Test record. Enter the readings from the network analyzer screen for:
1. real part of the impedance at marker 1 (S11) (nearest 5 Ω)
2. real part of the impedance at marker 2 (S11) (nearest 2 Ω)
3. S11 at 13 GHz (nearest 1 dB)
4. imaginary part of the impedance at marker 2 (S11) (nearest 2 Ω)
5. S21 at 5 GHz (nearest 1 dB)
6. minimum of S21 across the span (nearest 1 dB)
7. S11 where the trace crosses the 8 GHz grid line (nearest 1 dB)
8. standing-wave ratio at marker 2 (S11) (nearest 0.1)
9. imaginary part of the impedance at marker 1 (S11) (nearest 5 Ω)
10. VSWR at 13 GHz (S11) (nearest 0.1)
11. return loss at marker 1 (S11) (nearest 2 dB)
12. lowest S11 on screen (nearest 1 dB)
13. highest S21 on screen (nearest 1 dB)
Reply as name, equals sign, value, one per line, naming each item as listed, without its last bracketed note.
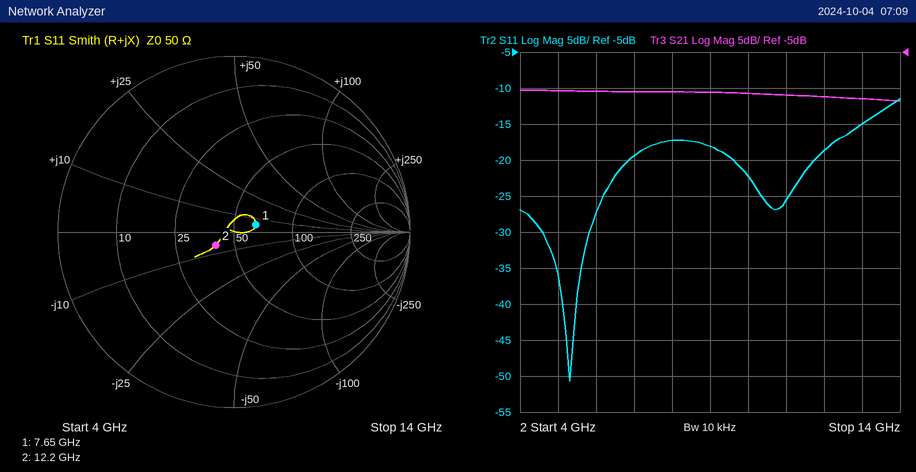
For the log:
real part of the impedance at marker 1 (S11) = 65 Ω
real part of the impedance at marker 2 (S11) = 40 Ω
S11 at 13 GHz = -15 dB
imaginary part of the impedance at marker 2 (S11) = -6 Ω
S21 at 5 GHz = -10 dB
minimum of S21 across the span = -12 dB
S11 where the trace crosses the 8 GHz grid line = -17 dB
standing-wave ratio at marker 2 (S11) = 1.3
imaginary part of the impedance at marker 1 (S11) = +5 Ω
VSWR at 13 GHz (S11) = 1.4
return loss at marker 1 (S11) = 18 dB
lowest S11 on screen = -51 dB
highest S21 on screen = -10 dB
